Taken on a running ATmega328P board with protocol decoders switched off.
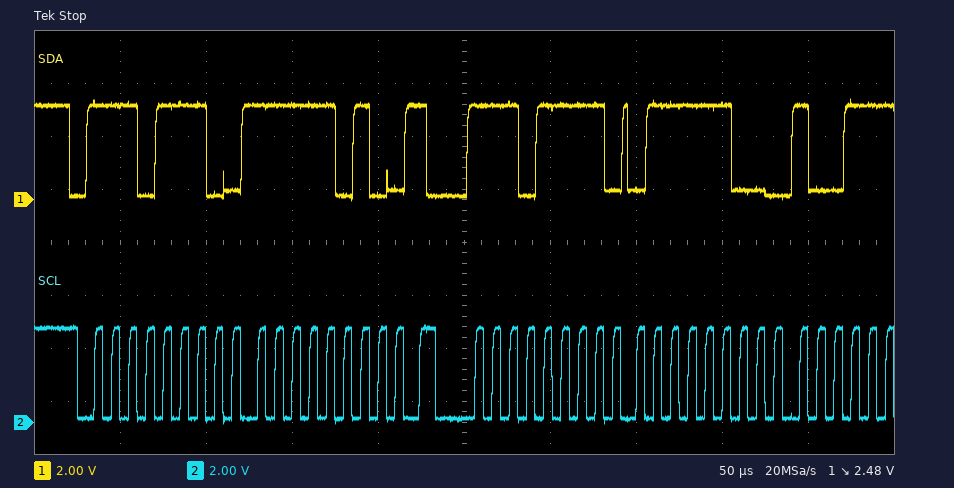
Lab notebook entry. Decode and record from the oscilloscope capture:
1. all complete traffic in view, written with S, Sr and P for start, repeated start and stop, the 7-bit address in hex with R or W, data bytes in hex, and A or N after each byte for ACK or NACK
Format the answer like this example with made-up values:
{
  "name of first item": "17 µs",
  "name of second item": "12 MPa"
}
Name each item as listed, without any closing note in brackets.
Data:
{
  "all complete traffic in view, written with S, Sr and P for start, repeated start and stop, the 7-bit address in hex with R or W, data bytes in hex, and A or N after each byte for ACK or NACK": "S 77W A FA A Sr 77R A 7C A"
}
